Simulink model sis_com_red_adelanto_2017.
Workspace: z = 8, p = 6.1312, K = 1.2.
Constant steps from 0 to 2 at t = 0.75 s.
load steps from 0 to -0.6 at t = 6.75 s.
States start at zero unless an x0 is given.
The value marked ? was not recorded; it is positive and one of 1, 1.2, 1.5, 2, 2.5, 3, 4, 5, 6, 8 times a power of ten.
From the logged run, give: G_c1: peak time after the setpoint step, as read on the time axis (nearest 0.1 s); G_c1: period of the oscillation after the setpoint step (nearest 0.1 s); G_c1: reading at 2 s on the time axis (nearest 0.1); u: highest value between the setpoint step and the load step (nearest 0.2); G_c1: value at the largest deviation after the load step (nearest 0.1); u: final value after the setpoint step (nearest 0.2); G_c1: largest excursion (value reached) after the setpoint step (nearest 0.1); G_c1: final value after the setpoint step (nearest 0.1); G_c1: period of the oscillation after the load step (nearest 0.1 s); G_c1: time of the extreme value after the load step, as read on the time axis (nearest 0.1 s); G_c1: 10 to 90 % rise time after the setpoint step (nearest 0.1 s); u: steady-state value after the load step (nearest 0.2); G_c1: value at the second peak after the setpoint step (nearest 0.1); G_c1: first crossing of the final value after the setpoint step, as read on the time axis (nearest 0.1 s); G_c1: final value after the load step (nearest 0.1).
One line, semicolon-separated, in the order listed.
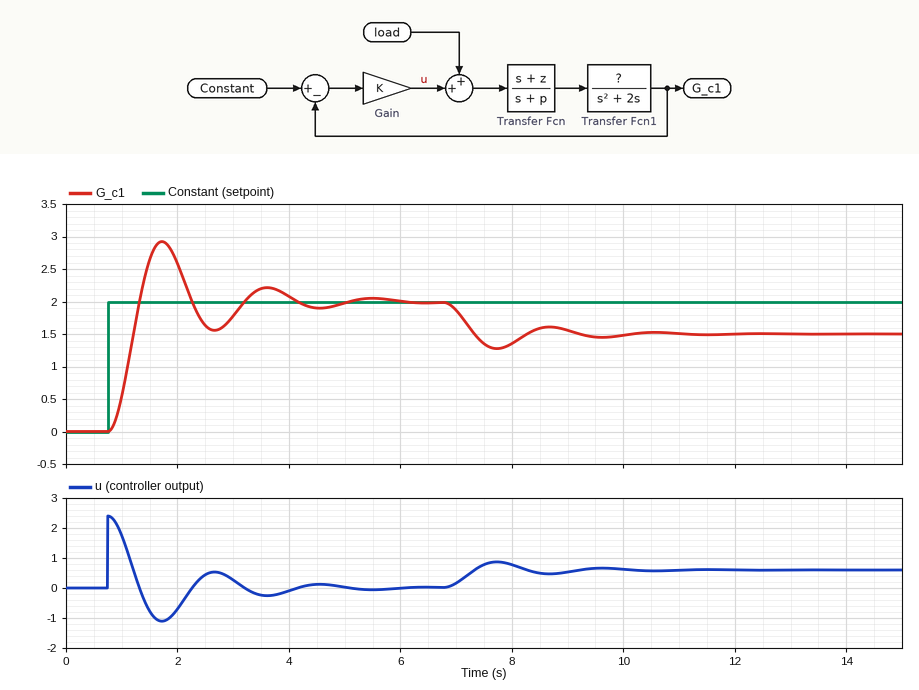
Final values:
1.7 s; 1.9 s; 2.6; 2.4; 1.3; 0.0; 2.9; 2.0; 1.9 s; 7.7 s; 0.4 s; 0.6; 2.2; 1.3 s; 1.5
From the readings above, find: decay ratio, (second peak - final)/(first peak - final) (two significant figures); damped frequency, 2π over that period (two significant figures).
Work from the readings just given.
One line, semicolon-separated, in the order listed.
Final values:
0.22; 3.3 rad/s
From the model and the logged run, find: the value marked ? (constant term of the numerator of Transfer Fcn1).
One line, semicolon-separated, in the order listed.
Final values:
8
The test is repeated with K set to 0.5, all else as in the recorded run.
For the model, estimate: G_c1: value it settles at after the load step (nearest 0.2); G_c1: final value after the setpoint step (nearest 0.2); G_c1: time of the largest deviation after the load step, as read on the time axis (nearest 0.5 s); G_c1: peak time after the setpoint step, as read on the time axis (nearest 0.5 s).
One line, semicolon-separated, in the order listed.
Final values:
0.8; 2.0; 8.5 s; 2.5 s
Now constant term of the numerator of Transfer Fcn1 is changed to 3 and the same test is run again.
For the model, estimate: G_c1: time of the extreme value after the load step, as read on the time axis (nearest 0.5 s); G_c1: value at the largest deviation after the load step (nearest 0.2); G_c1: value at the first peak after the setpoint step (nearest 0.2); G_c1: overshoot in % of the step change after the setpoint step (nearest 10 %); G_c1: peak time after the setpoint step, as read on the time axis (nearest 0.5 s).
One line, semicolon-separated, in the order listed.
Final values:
8.5 s; 1.4; 2.4; 20 %; 2.5 s
